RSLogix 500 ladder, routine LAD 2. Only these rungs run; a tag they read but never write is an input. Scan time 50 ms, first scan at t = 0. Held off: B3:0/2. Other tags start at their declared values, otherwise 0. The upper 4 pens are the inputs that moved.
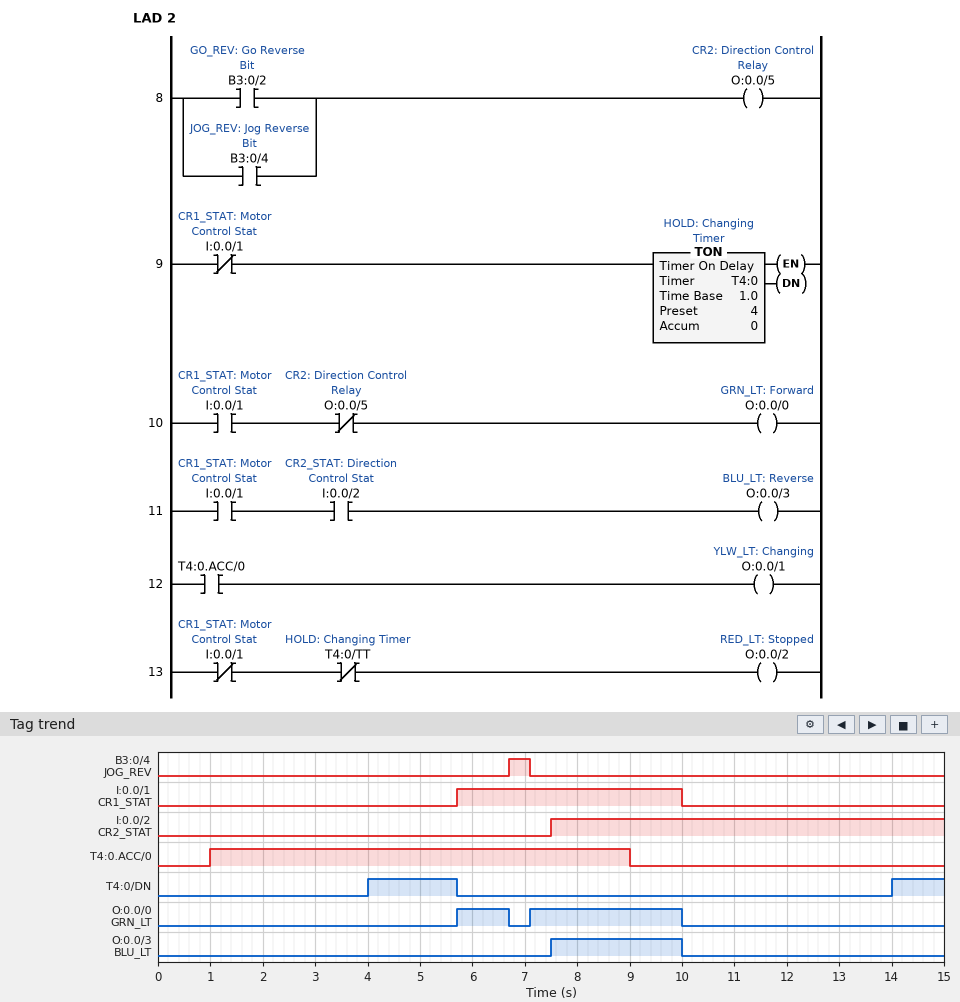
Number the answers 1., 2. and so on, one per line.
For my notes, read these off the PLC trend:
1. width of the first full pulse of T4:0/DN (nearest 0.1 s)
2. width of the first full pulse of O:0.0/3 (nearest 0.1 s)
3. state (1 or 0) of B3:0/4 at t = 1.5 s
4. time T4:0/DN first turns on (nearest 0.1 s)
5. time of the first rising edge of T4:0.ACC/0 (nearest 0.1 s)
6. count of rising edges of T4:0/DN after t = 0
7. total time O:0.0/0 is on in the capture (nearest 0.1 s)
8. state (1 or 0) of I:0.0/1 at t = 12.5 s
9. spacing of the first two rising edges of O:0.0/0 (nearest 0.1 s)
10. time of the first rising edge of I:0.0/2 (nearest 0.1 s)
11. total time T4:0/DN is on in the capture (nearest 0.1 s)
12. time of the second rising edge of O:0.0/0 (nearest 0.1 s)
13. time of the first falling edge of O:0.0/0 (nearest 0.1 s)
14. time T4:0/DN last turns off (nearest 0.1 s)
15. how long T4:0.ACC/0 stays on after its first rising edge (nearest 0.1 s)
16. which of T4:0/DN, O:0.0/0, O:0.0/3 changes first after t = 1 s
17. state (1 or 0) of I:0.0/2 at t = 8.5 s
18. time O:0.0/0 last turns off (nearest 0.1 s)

1. 1.7 s
2. 2.5 s
3. 0
4. 4.0 s
5. 1.0 s
6. 2
7. 3.9 s
8. 0
9. 1.4 s
10. 7.5 s
11. 2.7 s
12. 7.1 s
13. 6.7 s
14. 5.7 s
15. 8.0 s
16. T4:0/DN
17. 1
18. 10.0 s
